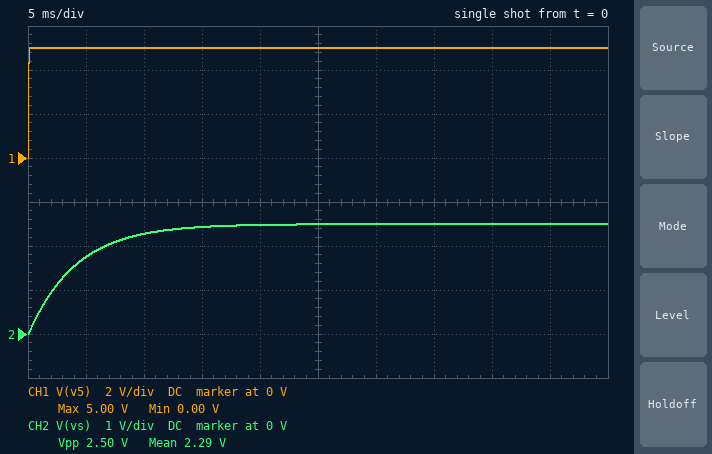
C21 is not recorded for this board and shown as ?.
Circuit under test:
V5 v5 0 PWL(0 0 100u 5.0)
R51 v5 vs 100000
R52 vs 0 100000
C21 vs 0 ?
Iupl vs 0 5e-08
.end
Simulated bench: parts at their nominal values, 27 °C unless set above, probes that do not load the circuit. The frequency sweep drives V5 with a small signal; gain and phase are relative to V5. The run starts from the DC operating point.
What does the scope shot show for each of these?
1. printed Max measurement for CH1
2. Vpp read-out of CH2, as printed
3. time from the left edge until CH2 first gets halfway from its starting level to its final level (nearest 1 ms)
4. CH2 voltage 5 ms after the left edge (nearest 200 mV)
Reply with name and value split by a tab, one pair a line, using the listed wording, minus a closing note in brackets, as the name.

printed Max measurement for CH1	5.00 V
Vpp read-out of CH2, as printed	2.50 V
time from the left edge until CH2 first gets halfway from its starting level to its final level	3 ms
CH2 voltage 5 ms after the left edge	1.8 V
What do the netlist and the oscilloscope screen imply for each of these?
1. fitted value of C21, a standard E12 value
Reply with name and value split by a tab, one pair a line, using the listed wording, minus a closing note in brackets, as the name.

fitted value of C21, a standard E12 value	82 nF
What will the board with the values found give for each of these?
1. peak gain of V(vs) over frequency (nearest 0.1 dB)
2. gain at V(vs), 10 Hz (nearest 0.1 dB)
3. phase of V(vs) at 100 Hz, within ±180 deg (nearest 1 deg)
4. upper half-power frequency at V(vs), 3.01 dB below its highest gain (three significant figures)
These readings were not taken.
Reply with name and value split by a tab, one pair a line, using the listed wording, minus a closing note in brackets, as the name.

peak gain of V(vs) over frequency	-6.0 dB
gain at V(vs), 10 Hz	-6.3 dB
phase of V(vs) at 100 Hz, within ±180 deg	-69 deg
upper half-power frequency at V(vs), 3.01 dB below its highest gain	38.8 Hz
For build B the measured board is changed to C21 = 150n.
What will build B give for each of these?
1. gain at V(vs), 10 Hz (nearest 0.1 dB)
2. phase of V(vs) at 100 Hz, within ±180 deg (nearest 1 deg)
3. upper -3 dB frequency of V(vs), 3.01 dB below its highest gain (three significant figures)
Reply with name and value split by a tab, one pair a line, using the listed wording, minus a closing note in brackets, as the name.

gain at V(vs), 10 Hz	-6.9 dB
phase of V(vs) at 100 Hz, within ±180 deg	-78 deg
upper -3 dB frequency of V(vs), 3.01 dB below its highest gain	21.2 Hz
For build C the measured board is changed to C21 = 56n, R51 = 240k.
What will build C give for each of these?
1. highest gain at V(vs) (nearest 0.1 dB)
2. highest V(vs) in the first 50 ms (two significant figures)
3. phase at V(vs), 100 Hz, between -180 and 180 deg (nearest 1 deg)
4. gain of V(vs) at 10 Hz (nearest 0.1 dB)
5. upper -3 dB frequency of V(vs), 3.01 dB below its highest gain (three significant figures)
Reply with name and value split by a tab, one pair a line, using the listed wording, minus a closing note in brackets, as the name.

highest gain at V(vs)	-10.6 dB
highest V(vs) in the first 50 ms	1.5 V
phase at V(vs), 100 Hz, between -180 and 180 deg	-68 deg
gain of V(vs) at 10 Hz	-10.9 dB
upper -3 dB frequency of V(vs), 3.01 dB below its highest gain	40.3 Hz
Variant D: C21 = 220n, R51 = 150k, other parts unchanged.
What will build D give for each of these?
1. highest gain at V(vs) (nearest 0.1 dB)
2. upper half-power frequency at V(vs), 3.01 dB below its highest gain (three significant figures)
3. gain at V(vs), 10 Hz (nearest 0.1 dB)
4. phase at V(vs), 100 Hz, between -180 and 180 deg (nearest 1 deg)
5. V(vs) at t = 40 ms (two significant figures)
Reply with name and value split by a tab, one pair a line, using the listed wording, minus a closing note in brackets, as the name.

highest gain at V(vs)	-8.0 dB
upper half-power frequency at V(vs), 3.01 dB below its highest gain	12.1 Hz
gain at V(vs), 10 Hz	-10.2 dB
phase at V(vs), 100 Hz, between -180 and 180 deg	-83 deg
V(vs) at t = 40 ms	1.9 V
